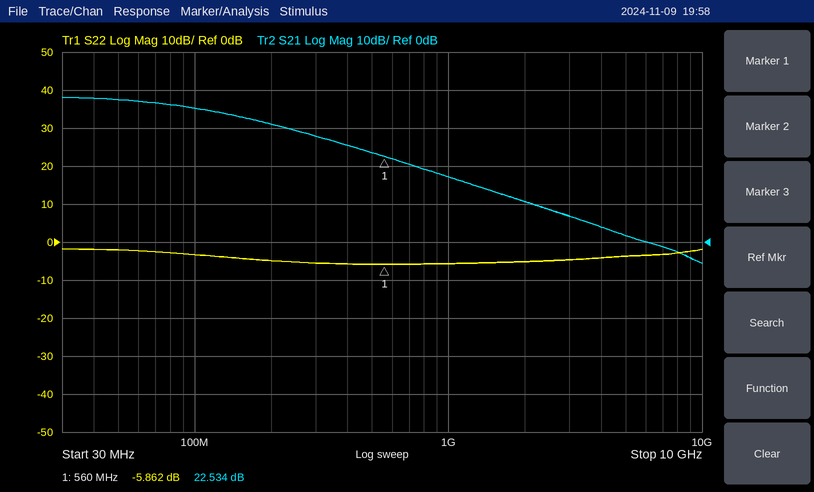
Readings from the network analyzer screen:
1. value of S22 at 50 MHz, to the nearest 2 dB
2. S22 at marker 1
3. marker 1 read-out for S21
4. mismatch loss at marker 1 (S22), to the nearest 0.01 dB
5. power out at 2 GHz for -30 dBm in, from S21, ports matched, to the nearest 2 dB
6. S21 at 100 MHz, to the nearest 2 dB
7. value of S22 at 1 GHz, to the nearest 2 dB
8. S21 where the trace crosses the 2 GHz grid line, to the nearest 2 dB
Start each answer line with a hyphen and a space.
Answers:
- -2 dB
- -5.862 dB
- 22.534 dB
- 1.30 dB
- -20 dBm
- 36 dB
- -6 dB
- 10 dB
